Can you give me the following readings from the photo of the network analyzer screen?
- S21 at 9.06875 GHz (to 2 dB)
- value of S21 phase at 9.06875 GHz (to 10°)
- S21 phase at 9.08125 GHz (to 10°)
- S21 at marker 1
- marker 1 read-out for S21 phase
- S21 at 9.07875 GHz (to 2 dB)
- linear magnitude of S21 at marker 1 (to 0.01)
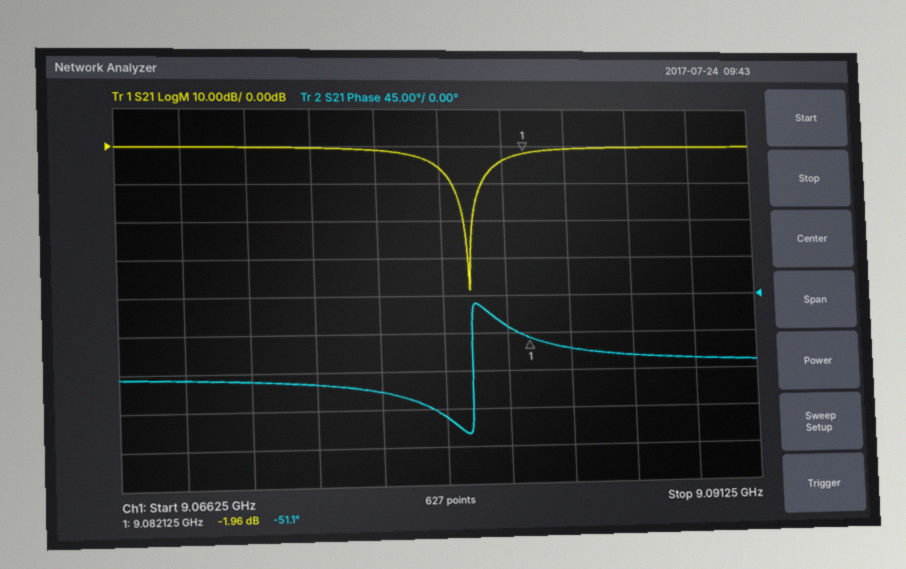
0 dB
-100°
-40°
-1.96 dB
-51.1°
-6 dB
0.80
